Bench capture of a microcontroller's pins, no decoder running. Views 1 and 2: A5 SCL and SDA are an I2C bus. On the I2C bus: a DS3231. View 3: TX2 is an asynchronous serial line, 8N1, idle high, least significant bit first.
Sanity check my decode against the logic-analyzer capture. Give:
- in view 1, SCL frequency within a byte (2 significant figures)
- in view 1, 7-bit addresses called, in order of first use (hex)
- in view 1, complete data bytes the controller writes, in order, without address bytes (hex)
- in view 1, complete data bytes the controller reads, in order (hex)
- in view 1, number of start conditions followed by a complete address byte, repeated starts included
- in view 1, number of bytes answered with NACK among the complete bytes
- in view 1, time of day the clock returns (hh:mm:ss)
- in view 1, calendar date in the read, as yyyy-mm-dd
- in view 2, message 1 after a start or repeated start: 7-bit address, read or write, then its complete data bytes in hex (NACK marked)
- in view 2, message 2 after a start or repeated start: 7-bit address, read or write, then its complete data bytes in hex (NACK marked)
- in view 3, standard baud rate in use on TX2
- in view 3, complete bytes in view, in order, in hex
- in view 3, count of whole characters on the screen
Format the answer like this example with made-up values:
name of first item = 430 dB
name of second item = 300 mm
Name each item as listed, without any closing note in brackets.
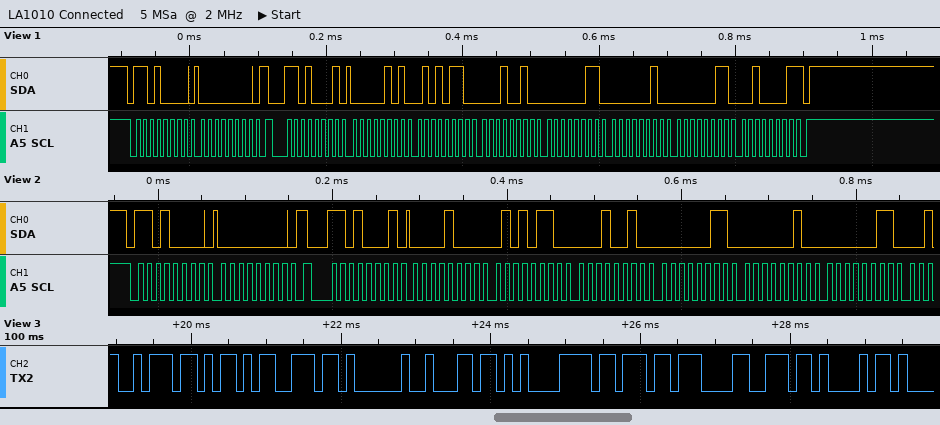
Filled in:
in view 1, SCL frequency within a byte = 100 kHz
in view 1, 7-bit addresses called, in order of first use = 0x68
in view 1, complete data bytes the controller writes, in order, without address bytes = 00
in view 1, complete data bytes the controller reads, in order = 05 56 12 03 02 03 21
in view 1, number of start conditions followed by a complete address byte, repeated starts included = 2
in view 1, number of bytes answered with NACK among the complete bytes = 1
in view 1, time of day the clock returns = 12:56:05
in view 1, calendar date in the read, as yyyy-mm-dd = 2021-03-02
in view 2, message 1 after a start or repeated start: 7-bit address, read or write, then its complete data bytes in hex = 0x68 write: 00
in view 2, message 2 after a start or repeated start: 7-bit address, read or write, then its complete data bytes in hex = 0x68 read: 08 56 12 03 02 03
in view 3, standard baud rate in use on TX2 = 9600 baud
in view 3, complete bytes in view, in order, in hex = BA AD 6E 20 6C E1 BB 87 6E 68
in view 3, count of whole characters on the screen = 10
